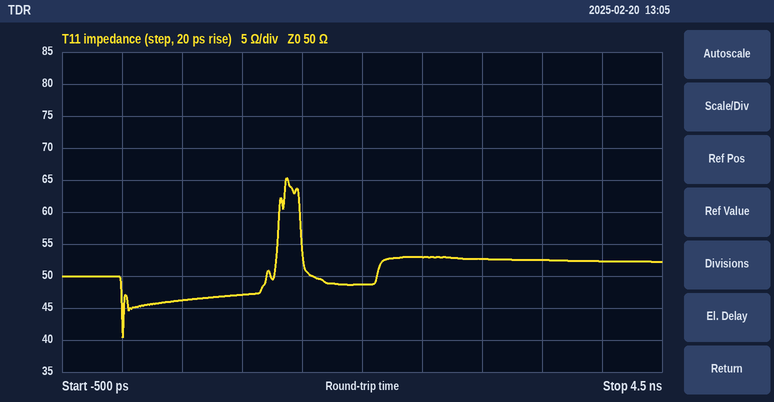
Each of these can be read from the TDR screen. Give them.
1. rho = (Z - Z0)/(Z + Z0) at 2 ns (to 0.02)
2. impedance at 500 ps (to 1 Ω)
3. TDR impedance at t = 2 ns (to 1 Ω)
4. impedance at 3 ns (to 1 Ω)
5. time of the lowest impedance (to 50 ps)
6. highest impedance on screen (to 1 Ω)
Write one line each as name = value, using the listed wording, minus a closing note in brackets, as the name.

rho = (Z - Z0)/(Z + Z0) at 2 ns = -0.02
impedance at 500 ps = 46 Ω
TDR impedance at t = 2 ns = 49 Ω
impedance at 3 ns = 53 Ω
time of the lowest impedance = 0 ps
highest impedance on screen = 65 Ω
